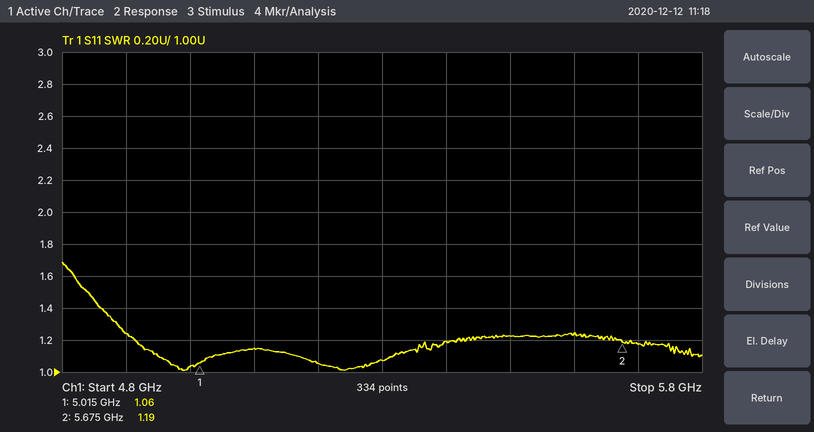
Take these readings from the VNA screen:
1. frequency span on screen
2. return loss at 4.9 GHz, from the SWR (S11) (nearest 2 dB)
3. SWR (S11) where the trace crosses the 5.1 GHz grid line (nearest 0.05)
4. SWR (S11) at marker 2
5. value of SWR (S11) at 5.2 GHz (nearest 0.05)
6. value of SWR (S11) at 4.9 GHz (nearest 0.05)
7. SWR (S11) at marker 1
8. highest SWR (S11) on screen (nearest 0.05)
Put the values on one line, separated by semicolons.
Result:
1 GHz; 20 dB; 1.15; 1.19; 1.05; 1.25; 1.06; 1.70
